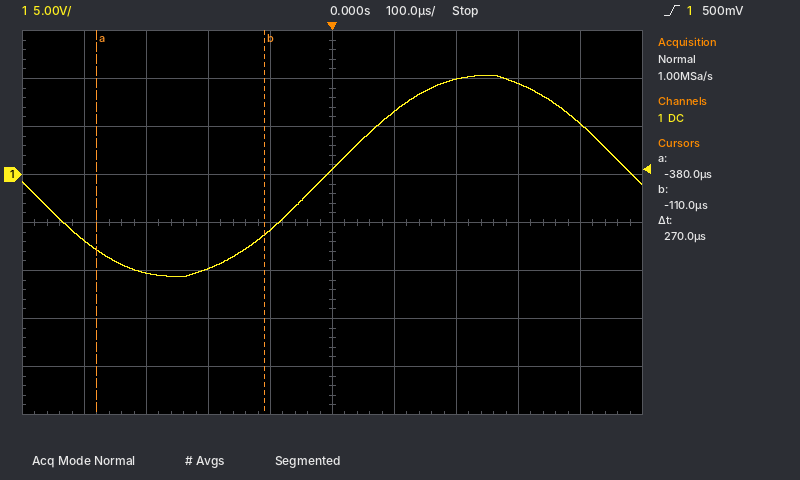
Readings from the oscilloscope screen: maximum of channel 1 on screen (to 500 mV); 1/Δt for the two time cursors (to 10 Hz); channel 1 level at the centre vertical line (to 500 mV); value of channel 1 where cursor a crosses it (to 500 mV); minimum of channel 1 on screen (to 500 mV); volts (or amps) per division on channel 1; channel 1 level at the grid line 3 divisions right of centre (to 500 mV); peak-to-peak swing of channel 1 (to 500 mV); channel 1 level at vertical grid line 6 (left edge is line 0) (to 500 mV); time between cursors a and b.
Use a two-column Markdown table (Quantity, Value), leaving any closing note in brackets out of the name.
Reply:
| Quantity | Value |
|---|---|
| maximum of channel 1 on screen | 10.5 V |
| 1/Δt for the two time cursors | 3.70 kHz |
| channel 1 level at the centre vertical line | 500 mV |
| value of channel 1 where cursor a crosses it | -8.0 V |
| minimum of channel 1 on screen | -10.5 V |
| volts (or amps) per division on channel 1 | 5 V |
| channel 1 level at the grid line 3 divisions right of centre | 9.5 V |
| peak-to-peak swing of channel 1 | 21.0 V |
| channel 1 level at vertical grid line 6 (left edge is line 0) | 6.5 V |
| time between cursors a and b | 270 µs |
